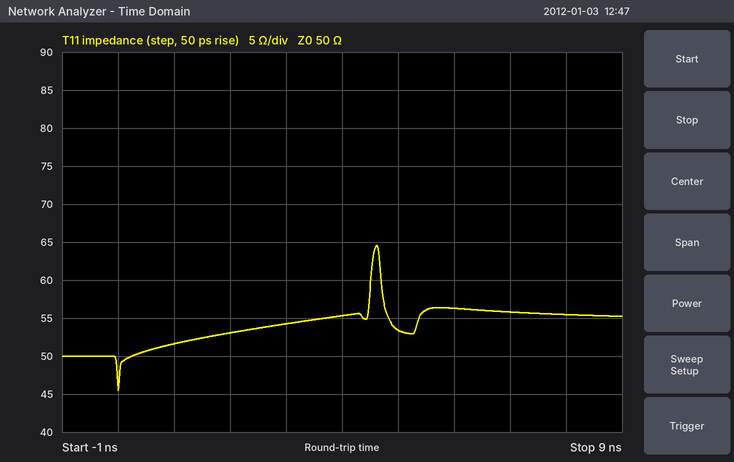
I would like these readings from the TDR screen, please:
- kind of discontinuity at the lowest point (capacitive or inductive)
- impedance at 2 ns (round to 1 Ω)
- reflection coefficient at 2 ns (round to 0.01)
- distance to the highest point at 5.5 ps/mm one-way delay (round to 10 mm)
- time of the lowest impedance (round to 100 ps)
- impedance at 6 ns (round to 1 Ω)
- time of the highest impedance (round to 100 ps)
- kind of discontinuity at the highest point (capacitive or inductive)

capacitive
53 Ω
+0.03
420 mm
0.0 ns
56 Ω
4.6 ns
inductive
